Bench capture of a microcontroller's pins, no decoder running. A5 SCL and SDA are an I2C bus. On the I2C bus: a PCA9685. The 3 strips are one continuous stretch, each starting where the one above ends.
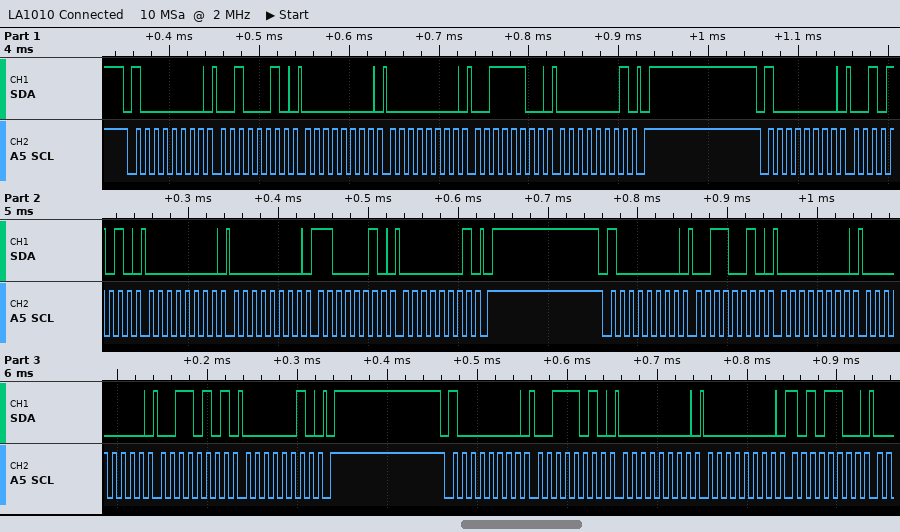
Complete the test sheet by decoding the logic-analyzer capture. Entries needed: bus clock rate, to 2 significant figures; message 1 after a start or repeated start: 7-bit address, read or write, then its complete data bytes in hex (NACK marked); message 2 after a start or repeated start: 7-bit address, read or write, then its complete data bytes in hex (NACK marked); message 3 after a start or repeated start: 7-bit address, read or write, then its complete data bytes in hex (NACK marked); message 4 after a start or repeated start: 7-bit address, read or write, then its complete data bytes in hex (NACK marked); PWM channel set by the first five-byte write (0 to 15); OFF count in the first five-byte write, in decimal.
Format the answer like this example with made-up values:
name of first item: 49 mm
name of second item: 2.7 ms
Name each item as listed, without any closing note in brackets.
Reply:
bus clock rate, to 2 significant figures: 100 kHz
message 1 after a start or repeated start: 7-bit address, read or write, then its complete data bytes in hex: 0x40 write: 22 00 00 3C 01
message 2 after a start or repeated start: 7-bit address, read or write, then its complete data bytes in hex: 0x40 write: 2A 00 00 C2 01
message 3 after a start or repeated start: 7-bit address, read or write, then its complete data bytes in hex: 0x40 write: 32 00 00 35 02
message 4 after a start or repeated start: 7-bit address, read or write, then its complete data bytes in hex: 0x40 write: 3A 00 00 AC
PWM channel set by the first five-byte write: 7
OFF count in the first five-byte write, in decimal: 316
